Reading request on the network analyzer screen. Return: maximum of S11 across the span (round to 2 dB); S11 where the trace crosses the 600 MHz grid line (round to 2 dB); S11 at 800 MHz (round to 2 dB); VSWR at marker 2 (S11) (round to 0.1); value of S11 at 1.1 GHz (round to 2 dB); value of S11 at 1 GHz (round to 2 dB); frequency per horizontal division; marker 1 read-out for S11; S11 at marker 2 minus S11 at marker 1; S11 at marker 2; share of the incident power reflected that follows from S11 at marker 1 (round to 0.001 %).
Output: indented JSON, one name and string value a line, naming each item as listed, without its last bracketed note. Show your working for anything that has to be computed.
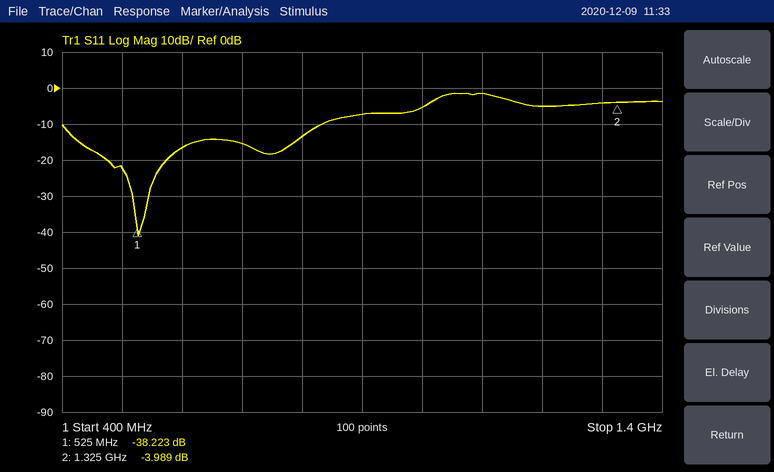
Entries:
{
  "maximum of S11 across the span": "-2 dB",
  "S11 where the trace crosses the 600 MHz grid line": "-16 dB",
  "S11 at 800 MHz": "-14 dB",
  "VSWR at marker 2 (S11)": "(1 + 0.6318)/(1 − 0.6318) ≈ 4.4",
  "value of S11 at 1.1 GHz": "-2 dB",
  "value of S11 at 1 GHz": "-6 dB",
  "frequency per horizontal division": "100 MHz",
  "marker 1 read-out for S11": "-38.223 dB",
  "S11 at marker 2 minus S11 at marker 1": "-3.989 − (-38.223) = 34.234 dB",
  "S11 at marker 2": "-3.989 dB",
  "share of the incident power reflected that follows from S11 at marker 1": "10^(-38.223/10) ≈ 0.015 %"
}
